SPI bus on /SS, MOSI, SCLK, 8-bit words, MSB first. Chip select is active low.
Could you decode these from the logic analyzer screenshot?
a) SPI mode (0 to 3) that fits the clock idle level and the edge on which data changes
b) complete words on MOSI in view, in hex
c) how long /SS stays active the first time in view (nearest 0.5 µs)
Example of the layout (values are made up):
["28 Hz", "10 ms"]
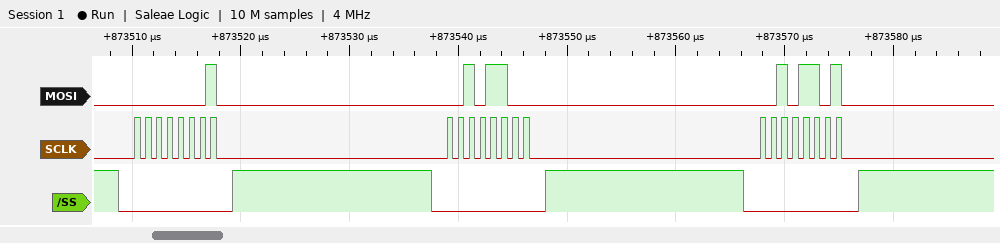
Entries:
["0", "01, 2C, 2D", "10.5 µs"]
